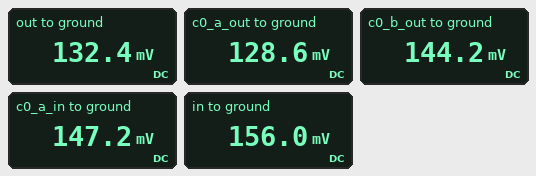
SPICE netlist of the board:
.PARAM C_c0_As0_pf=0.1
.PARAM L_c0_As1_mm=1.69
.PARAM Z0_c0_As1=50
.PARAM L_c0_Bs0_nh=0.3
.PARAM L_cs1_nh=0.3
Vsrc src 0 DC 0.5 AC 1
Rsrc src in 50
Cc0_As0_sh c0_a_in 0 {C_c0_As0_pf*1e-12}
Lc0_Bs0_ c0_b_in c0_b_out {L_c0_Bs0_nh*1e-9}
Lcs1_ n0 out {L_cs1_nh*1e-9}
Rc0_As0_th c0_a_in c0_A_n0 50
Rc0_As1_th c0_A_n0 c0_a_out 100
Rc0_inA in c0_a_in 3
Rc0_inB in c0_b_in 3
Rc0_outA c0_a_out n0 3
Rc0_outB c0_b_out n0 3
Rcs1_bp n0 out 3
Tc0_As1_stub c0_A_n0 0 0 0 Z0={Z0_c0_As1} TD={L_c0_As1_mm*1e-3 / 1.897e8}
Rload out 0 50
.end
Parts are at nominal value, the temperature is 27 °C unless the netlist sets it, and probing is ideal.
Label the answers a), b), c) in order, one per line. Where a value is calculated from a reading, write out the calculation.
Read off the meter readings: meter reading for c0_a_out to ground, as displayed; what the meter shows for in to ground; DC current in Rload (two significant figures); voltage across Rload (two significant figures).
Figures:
a) 128.6 mV
b) 156.0 mV
c) (132.4 mV) / 50 Ω = 2.6 mA
d) 132.4 mV = 130 mV
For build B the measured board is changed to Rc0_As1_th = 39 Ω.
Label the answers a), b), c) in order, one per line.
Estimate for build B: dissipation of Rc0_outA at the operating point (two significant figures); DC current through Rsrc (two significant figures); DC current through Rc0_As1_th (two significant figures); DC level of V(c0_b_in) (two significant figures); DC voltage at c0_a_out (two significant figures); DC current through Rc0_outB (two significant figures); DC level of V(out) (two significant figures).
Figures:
a) 20 µW
b) 7.3 mA
c) 2.6 mA
d) 120 mV
e) 100 mV
f) 4.7 mA
g) 110 mV
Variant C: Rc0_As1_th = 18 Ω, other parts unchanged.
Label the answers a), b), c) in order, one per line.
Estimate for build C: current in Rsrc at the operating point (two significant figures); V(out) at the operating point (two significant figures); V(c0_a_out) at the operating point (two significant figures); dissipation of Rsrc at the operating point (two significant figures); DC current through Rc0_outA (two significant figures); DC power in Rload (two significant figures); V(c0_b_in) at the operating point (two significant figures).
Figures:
a) 7.7 mA
b) 82 mV
c) 70 mV
d) 3.0 mW
e) 3.9 mA
f) 130 µW
g) 98 mV
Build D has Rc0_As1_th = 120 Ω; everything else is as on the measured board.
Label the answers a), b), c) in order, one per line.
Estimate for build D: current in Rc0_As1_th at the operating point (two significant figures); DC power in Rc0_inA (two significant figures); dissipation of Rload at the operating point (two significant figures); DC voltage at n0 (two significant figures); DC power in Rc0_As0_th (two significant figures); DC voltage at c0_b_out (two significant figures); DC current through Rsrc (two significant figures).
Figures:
a) 1.1 mA
b) 27 µW
c) 370 µW
d) 140 mV
e) 450 µW
f) 150 mV
g) 6.8 mA
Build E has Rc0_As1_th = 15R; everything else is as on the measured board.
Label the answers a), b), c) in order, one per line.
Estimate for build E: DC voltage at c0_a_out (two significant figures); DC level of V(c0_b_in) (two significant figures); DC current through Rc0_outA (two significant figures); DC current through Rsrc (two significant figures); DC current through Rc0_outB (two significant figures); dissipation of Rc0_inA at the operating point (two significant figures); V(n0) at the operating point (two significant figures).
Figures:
a) 63 mV
b) 93 mV
c) 4.2 mA
d) 7.8 mA
e) 5.7 mA
f) 13 µW
g) 76 mV
